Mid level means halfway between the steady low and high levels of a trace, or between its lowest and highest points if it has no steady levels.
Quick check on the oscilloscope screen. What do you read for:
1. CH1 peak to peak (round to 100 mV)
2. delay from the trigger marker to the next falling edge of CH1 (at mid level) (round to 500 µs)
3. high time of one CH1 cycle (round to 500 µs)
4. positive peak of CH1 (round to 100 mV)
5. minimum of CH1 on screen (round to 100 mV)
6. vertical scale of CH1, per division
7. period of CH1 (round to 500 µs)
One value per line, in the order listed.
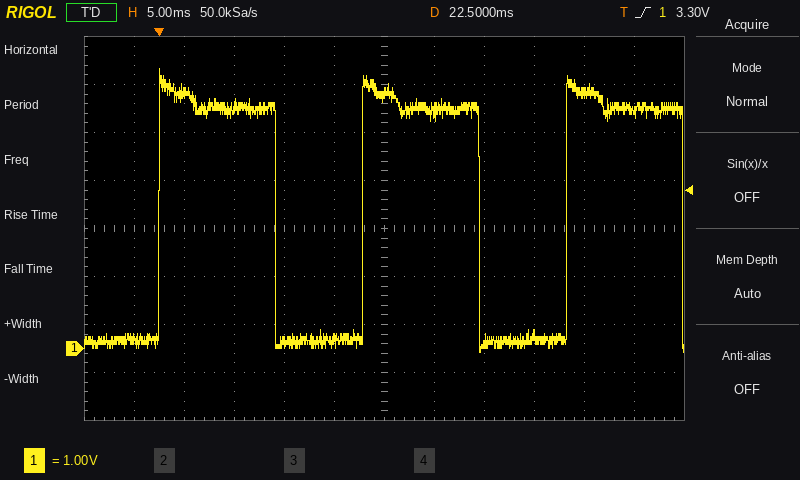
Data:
5.9 V
11.5 ms
11.5 ms
5.8 V
-100 mV
1 V
20.5 ms
